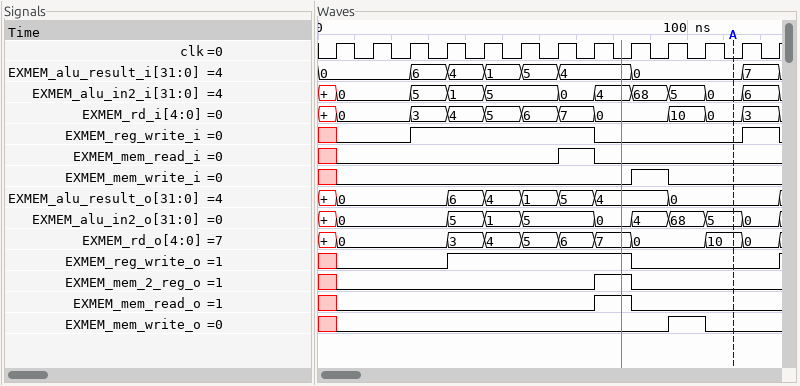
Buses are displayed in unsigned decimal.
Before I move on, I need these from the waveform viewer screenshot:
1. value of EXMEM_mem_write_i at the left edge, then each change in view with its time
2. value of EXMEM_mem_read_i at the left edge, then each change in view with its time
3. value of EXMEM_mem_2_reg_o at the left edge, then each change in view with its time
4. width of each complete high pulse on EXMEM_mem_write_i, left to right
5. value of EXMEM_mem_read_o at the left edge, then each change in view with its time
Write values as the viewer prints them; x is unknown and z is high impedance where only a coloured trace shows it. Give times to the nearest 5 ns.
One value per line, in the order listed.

x, 0 at 5 ns, 1 at 85 ns, 0 at 95 ns
x, 0 at 5 ns, 1 at 65 ns, 0 at 75 ns
x, 0 at 5 ns, 1 at 75 ns, 0 at 85 ns
10 ns
x, 0 at 5 ns, 1 at 75 ns, 0 at 85 ns
